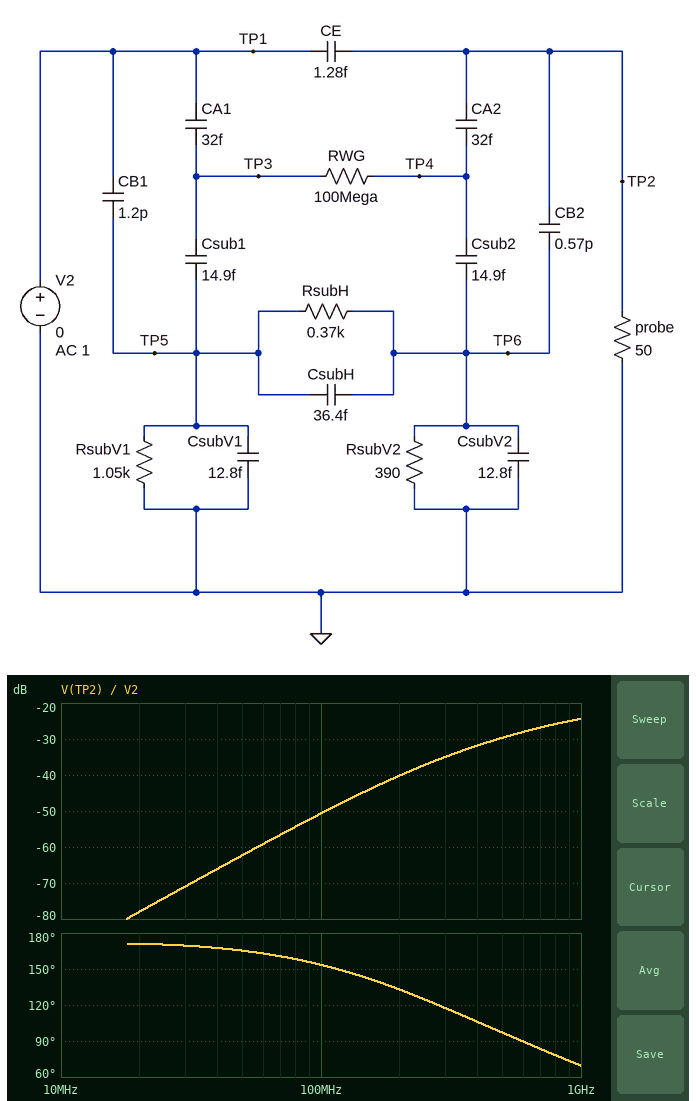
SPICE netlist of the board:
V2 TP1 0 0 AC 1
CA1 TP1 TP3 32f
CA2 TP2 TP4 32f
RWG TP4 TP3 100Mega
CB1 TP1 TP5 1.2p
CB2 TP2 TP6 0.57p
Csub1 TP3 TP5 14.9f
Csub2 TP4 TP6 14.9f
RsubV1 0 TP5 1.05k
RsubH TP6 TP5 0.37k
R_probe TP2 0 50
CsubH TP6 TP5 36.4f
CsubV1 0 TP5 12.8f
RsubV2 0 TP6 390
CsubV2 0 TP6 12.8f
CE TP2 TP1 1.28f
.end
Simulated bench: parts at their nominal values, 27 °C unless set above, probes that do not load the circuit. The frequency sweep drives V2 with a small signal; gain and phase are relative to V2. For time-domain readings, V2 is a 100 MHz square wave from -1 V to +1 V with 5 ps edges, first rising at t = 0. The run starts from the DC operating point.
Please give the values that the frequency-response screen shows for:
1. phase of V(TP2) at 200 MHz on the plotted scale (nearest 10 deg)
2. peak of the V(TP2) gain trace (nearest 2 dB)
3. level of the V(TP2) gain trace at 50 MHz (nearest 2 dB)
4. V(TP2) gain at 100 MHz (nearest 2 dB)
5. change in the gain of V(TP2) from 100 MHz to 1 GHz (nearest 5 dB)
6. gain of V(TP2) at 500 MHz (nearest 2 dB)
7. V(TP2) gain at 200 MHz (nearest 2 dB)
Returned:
130 deg
-24 dB
-62 dB
-50 dB
25 dB
-30 dB
-40 dB
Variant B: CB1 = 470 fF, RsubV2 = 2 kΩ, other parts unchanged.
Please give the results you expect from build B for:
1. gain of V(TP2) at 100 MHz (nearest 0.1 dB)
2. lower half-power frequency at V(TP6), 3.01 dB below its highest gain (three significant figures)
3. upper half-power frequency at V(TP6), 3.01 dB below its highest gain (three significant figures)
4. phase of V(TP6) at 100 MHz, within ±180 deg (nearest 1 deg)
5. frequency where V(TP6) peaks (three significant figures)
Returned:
-50.3 dB
164 MHz
2.06 GHz
61 deg
563 MHz
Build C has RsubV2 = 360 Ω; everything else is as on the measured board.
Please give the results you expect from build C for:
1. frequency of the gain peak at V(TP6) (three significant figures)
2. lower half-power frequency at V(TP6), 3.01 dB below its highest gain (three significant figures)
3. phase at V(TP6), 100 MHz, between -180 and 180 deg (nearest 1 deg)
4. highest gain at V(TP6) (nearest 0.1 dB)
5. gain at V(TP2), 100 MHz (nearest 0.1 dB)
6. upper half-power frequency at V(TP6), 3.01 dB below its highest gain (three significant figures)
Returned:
589 MHz
194 MHz
66 deg
-9.1 dB
-51.2 dB
1.89 GHz
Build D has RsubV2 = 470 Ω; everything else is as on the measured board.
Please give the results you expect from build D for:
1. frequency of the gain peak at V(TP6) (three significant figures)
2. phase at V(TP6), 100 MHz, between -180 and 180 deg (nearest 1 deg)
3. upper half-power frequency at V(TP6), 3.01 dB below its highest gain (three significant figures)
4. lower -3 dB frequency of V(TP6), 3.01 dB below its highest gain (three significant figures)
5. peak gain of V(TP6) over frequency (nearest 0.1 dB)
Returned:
536 MHz
63 deg
1.72 GHz
175 MHz
-8.2 dB
